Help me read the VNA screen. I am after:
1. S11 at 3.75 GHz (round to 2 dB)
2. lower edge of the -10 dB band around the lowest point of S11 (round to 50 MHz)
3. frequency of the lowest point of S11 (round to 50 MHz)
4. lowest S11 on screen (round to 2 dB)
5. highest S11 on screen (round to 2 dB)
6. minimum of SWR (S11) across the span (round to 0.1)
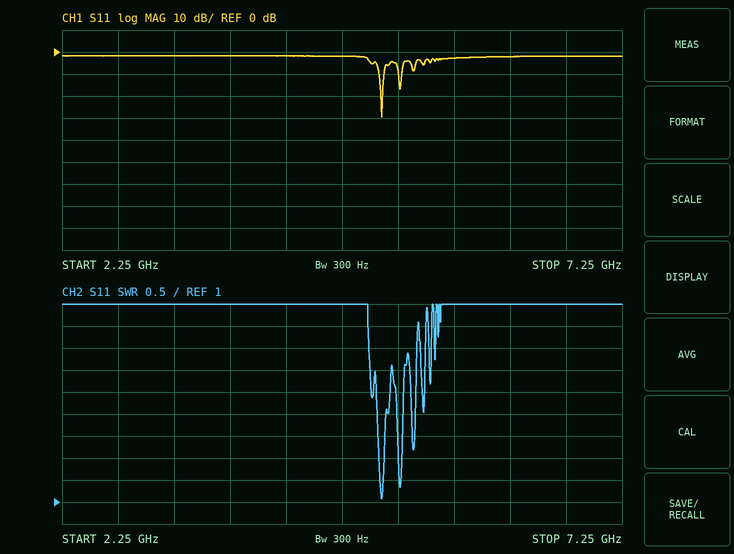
-2 dB
5.10 GHz
5.10 GHz
-30 dB
-2 dB
1.1
